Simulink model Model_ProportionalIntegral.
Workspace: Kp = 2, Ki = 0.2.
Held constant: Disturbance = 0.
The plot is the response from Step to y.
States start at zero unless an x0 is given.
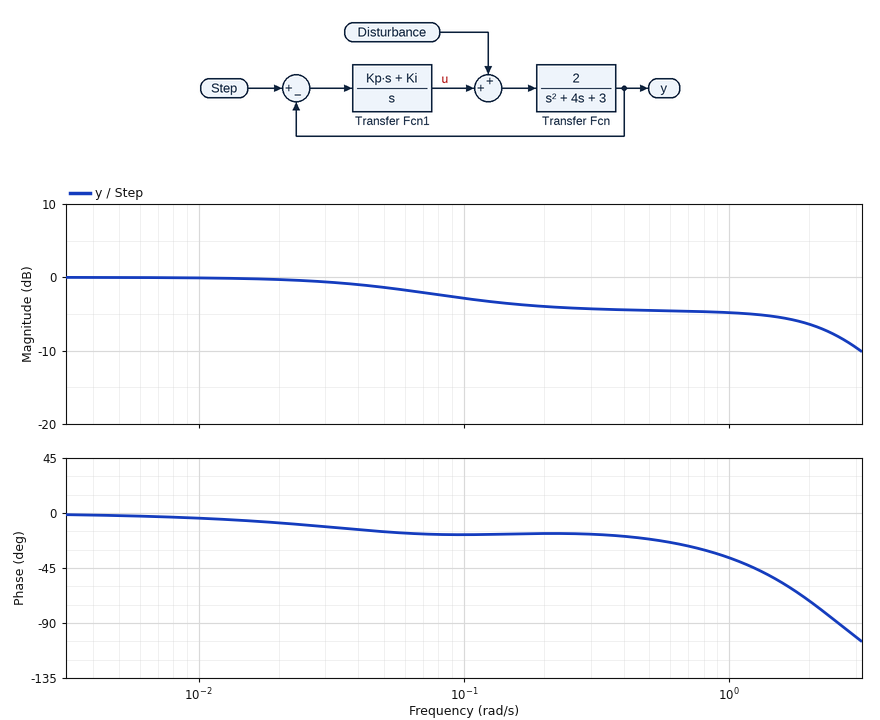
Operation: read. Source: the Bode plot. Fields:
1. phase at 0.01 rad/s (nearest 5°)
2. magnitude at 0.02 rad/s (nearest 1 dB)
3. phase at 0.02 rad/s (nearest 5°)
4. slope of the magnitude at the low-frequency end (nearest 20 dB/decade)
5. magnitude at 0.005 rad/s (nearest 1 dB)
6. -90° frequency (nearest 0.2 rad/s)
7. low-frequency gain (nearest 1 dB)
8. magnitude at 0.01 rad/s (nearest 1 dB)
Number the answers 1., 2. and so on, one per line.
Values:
1. -5°
2. 0 dB
3. -10°
4. 0 dB/decade
5. 0 dB
6. 2.6 rad/s
7. 0 dB
8. 0 dB
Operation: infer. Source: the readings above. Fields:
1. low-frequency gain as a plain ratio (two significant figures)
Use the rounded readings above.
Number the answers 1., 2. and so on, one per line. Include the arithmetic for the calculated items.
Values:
1. 10^(0 / 20) = 1.0
